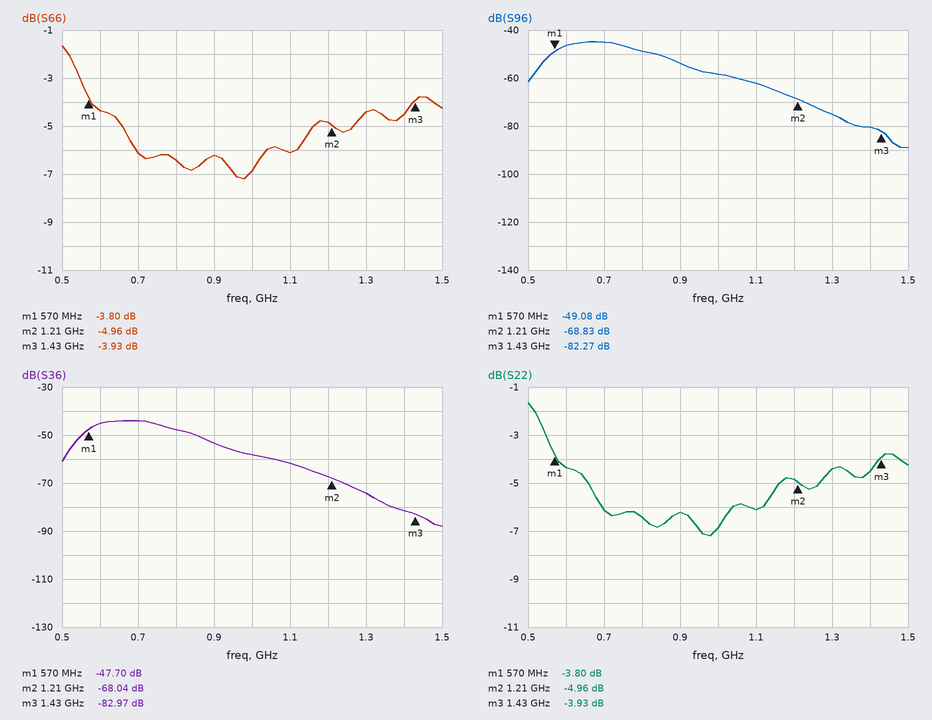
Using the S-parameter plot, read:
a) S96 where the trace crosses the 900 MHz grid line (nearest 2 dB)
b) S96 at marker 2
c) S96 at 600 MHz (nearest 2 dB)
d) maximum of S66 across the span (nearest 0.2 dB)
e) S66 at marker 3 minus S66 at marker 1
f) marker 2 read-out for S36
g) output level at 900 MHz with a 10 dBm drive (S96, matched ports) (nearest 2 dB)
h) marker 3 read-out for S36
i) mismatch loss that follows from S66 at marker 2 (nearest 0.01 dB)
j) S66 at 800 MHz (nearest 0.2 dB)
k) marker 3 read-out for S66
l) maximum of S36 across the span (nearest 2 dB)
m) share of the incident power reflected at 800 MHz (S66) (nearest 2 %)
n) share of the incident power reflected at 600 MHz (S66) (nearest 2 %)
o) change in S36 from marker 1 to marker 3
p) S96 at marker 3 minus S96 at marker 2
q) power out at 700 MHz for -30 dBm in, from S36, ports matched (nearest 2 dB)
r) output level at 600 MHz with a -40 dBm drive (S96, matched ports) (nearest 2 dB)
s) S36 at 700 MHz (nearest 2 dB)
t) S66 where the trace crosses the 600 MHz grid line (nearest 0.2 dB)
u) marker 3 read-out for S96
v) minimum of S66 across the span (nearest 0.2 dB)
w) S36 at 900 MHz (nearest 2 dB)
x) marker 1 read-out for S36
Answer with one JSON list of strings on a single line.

["-54 dB", "-68.83 dB", "-46 dB", "-1.6 dB", "-0.13 dB", "-68.04 dB", "-44 dBm", "-82.97 dB", "1.67 dB", "-6.4 dB", "-3.93 dB", "-44 dB", "22 %", "36 %", "-35.27 dB", "-13.44 dB", "-74 dBm", "-86 dBm", "-44 dB", "-4.4 dB", "-82.27 dB", "-7.2 dB", "-54 dB", "-47.70 dB"]
